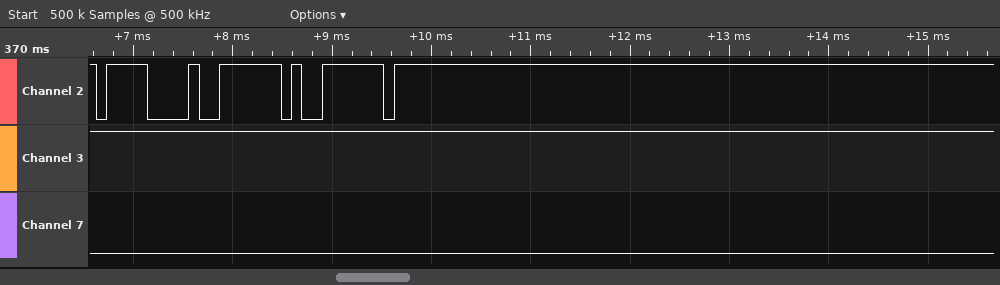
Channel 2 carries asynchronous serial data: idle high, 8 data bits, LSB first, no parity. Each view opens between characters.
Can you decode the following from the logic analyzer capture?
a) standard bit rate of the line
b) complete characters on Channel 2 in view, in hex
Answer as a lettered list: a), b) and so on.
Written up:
a) 9600 baud
b) 0F, 7E, 7E
